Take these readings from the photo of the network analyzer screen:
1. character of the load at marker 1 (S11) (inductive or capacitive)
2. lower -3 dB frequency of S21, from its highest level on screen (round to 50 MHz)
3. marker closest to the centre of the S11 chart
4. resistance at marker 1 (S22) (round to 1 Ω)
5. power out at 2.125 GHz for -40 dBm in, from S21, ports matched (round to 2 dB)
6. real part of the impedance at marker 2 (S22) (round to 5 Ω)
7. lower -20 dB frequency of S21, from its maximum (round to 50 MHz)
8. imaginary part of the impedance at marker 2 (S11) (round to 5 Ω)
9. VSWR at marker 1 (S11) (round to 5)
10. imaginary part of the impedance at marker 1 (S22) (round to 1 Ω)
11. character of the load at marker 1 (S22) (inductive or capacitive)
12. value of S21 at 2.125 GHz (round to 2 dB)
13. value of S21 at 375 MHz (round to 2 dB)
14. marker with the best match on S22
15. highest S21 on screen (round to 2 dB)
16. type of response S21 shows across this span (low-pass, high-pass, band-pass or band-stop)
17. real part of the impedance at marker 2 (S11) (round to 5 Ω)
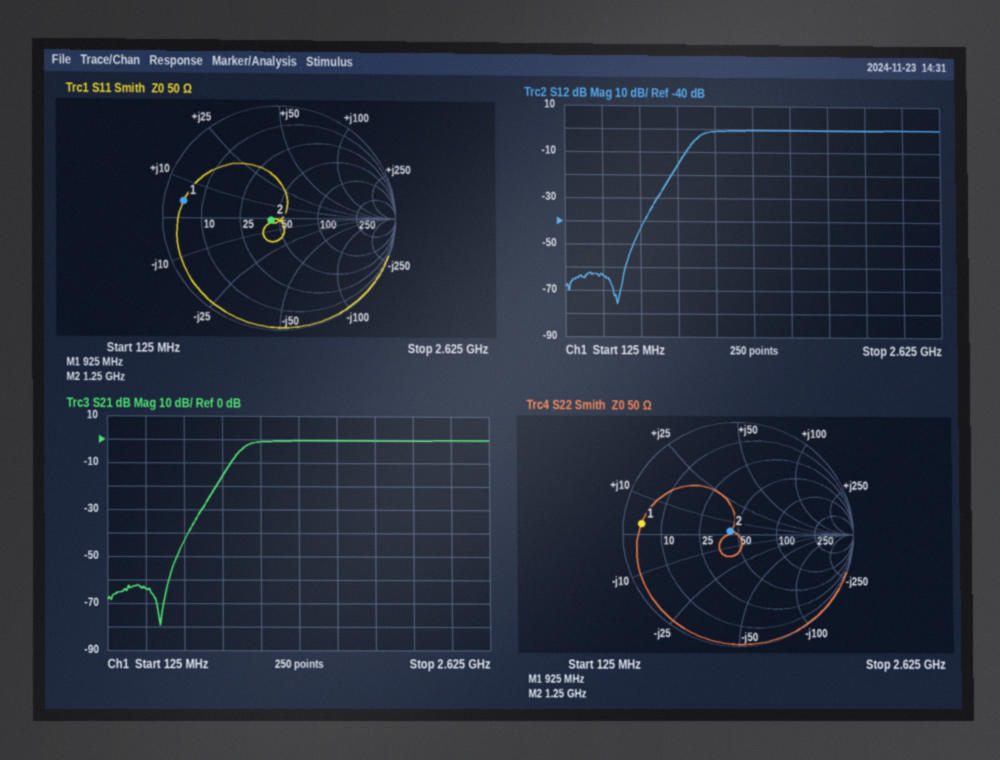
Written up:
inductive
1.00 GHz
marker 2
4 Ω
-40 dBm
45 Ω
850 MHz
0 Ω
10
+3 Ω
inductive
0 dB
-64 dB
marker 2
0 dB
high-pass
45 Ω
